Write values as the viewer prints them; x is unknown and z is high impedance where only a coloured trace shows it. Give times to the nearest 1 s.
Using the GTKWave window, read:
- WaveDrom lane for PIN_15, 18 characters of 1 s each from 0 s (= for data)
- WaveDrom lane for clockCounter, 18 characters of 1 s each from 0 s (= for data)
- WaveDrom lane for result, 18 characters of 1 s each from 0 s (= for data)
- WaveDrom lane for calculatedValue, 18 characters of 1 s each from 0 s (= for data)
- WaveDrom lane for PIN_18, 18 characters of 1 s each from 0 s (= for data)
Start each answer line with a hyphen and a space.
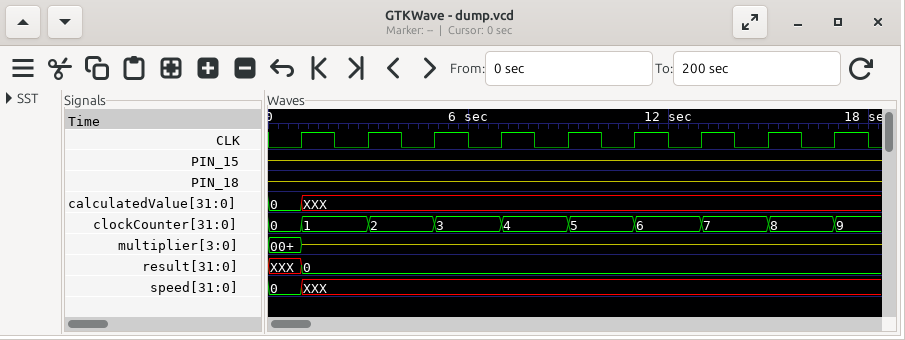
- {name: 'PIN_15', wave: 'z.................'}
- {name: 'clockCounter', wave: '==.=.=.=.=.=.=.=.=', data: '0 1 2 3 4 5 6 7 8 9'}
- {name: 'result', wave: 'x=................', data: '0'}
- {name: 'calculatedValue', wave: '=x................', data: '0'}
- {name: 'PIN_18', wave: 'z.................'}
